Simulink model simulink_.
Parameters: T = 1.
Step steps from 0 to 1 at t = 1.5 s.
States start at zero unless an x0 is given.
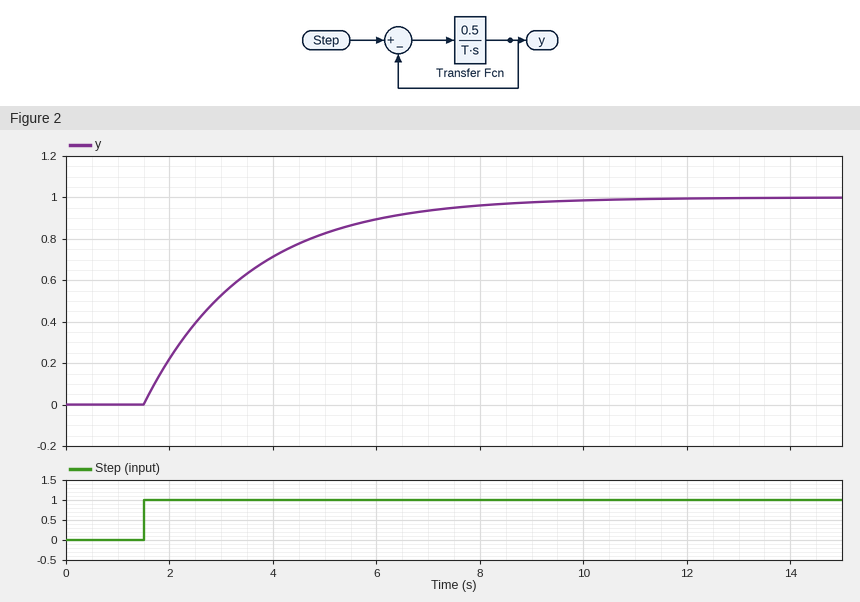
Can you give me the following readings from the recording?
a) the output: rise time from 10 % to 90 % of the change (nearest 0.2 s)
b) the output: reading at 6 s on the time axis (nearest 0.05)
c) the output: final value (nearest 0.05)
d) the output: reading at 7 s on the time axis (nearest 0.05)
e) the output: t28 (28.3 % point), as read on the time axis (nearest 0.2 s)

4.4 s
0.90
1.00
0.95
2.2 s
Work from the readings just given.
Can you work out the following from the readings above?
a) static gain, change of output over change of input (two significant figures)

1.0
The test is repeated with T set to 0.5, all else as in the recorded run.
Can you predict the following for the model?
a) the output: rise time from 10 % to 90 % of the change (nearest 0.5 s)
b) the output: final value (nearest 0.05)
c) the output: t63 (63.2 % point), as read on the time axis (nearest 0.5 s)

2.0 s
1.00
2.5 s
